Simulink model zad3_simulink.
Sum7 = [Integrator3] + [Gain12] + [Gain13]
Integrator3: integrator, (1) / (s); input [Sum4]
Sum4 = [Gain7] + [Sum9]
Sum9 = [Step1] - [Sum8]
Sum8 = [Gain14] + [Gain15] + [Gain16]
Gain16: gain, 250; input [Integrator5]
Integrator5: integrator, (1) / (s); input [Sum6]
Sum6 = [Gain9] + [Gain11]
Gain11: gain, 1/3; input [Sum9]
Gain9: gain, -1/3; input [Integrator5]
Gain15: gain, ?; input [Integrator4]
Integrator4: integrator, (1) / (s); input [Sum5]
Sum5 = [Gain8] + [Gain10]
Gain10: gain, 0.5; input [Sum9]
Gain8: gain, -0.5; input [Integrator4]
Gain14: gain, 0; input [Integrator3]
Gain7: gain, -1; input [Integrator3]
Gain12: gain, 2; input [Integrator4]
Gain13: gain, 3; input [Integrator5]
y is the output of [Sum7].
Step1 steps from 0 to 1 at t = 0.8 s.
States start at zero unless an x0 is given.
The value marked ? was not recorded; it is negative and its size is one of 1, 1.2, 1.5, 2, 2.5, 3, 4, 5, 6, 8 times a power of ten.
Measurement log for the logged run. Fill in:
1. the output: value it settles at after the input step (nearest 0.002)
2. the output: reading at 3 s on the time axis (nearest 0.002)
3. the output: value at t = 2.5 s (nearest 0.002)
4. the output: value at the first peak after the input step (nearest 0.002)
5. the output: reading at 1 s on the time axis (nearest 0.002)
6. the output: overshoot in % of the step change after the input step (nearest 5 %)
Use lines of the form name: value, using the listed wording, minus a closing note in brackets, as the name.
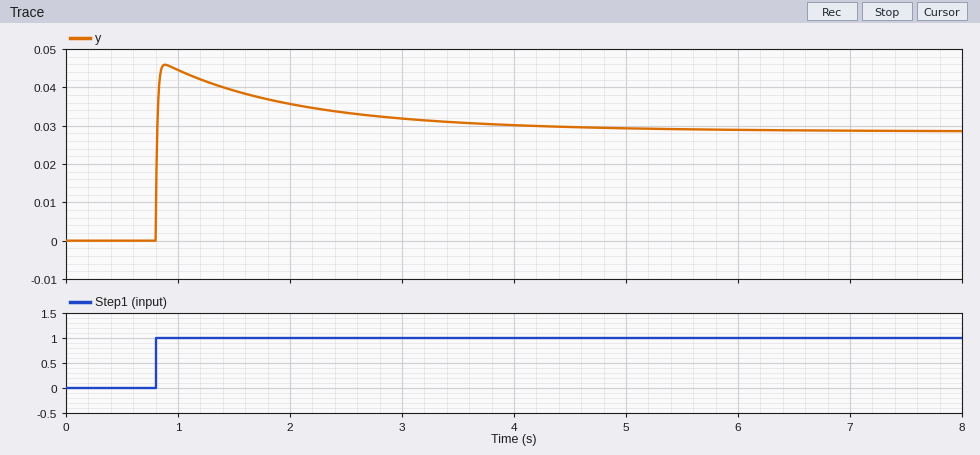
the output: value it settles at after the input step: 0.028
the output: reading at 3 s on the time axis: 0.032
the output: value at t = 2.5 s: 0.034
the output: value at the first peak after the input step: 0.046
the output: reading at 1 s on the time axis: 0.044
the output: overshoot in % of the step change after the input step: 60 %
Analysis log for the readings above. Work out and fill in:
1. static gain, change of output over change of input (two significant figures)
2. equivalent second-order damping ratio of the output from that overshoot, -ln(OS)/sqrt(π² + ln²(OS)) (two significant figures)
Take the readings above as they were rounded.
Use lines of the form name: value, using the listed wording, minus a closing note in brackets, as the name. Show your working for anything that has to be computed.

static gain, change of output over change of input: (0.028 - 0) / (1 - 0) = 0.028
equivalent second-order damping ratio of the output from that overshoot, -ln(OS)/sqrt(π² + ln²(OS)): ln(0.6) = -0.511; 0.511 / sqrt(9.870 + 0.261) = 0.16
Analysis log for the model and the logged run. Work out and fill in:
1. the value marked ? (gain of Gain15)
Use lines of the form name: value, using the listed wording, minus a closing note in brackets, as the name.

the value marked ?: -40
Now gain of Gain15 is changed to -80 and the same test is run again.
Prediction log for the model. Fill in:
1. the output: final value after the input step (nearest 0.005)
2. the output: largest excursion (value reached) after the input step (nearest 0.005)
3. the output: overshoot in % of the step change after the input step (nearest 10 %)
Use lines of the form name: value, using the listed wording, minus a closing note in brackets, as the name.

the output: final value after the input step: 0.035
the output: largest excursion (value reached) after the input step: 0.065
the output: overshoot in % of the step change after the input step: 90 %
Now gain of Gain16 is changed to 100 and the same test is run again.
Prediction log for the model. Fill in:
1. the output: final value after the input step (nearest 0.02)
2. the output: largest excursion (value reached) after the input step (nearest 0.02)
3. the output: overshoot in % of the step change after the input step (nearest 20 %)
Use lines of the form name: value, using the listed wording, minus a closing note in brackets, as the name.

the output: final value after the input step: 0.10
the output: largest excursion (value reached) after the input step: 0.20
the output: overshoot in % of the step change after the input step: 100 %
